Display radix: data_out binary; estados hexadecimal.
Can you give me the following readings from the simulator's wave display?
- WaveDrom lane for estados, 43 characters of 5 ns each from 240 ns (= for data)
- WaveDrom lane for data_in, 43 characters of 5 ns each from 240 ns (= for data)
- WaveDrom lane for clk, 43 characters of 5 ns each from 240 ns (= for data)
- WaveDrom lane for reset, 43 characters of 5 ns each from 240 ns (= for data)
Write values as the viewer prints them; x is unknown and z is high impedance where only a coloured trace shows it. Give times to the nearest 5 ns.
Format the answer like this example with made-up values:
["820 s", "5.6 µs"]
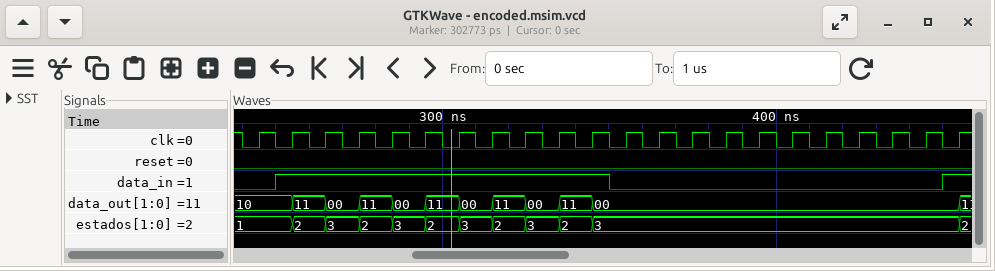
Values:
["{name: 'estados', wave: '=..=.=.=.=.=.=.=.=.=.=.....................', data: '1 2 3 2 3 2 3 2 3 2 3'}", "{name: 'data_in', wave: '0.1...................0...................1'}", "{name: 'clk', wave: '0101010101010101010101010101010101010101010'}", "{name: 'reset', wave: '0..........................................'}"]
